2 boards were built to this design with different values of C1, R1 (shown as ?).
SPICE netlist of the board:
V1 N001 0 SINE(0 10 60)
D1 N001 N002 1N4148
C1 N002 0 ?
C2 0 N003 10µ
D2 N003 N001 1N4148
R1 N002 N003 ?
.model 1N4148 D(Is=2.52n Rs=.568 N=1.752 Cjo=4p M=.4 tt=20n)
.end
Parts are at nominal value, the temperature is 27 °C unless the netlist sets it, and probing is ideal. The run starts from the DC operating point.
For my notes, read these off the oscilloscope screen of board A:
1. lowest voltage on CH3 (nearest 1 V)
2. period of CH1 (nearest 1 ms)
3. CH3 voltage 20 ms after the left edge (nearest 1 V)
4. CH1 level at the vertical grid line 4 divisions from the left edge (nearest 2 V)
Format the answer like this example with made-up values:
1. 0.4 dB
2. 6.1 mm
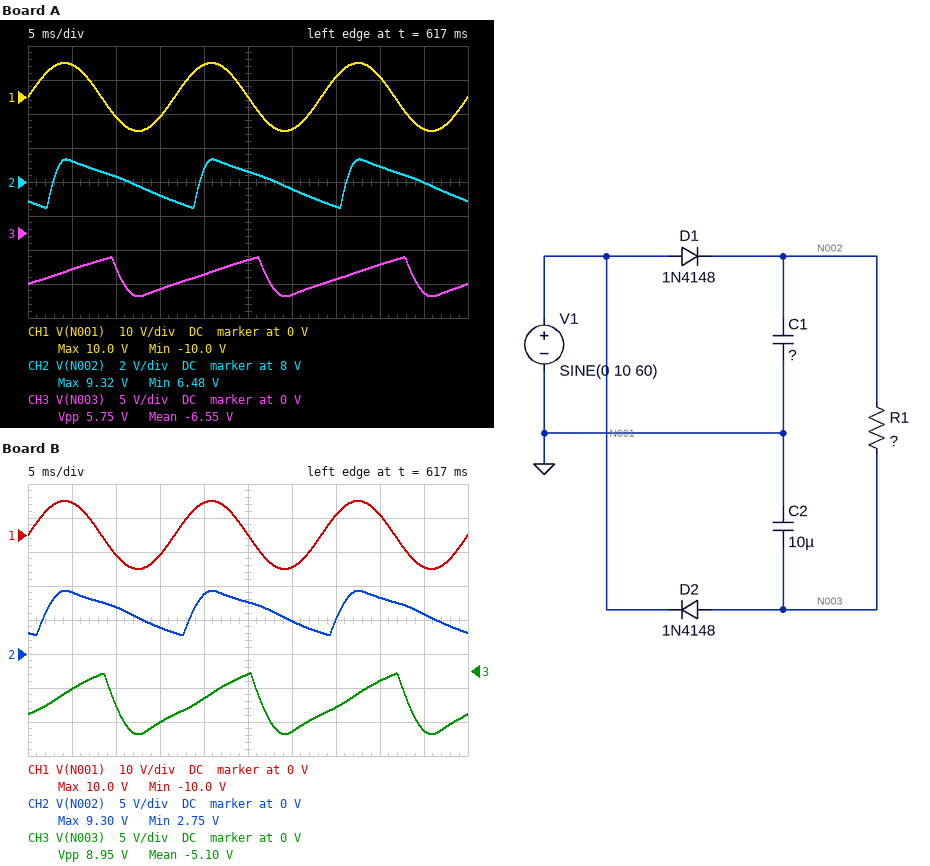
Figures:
1. -9 V
2. 17 ms
3. -6 V
4. 10 V
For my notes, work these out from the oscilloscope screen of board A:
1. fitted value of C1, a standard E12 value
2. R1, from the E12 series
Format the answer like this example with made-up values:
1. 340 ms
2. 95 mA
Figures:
1. 22 µF
2. 3.3 kΩ
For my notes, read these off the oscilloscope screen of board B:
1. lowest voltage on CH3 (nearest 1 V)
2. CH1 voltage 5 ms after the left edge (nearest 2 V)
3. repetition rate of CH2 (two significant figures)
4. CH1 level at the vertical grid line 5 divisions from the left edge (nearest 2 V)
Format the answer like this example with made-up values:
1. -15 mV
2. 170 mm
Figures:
1. -9 V
2. 10 V
3. 60 Hz
4. 0 V
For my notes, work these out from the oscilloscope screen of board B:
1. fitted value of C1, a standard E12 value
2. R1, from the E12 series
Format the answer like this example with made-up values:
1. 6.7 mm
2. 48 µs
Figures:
1. 15 µF
2. 1.5 kΩ
